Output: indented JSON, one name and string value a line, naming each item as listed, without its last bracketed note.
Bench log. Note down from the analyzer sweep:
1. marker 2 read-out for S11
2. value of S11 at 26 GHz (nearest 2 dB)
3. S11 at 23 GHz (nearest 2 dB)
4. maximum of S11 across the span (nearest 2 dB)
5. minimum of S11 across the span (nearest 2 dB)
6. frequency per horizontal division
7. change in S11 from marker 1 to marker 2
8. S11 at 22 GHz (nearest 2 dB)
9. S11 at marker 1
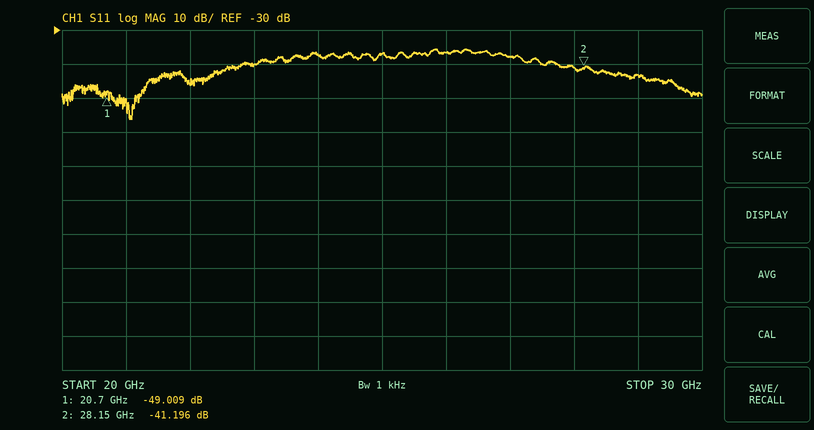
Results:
{
  "marker 2 read-out for S11": "-41.196 dB",
  "value of S11 at 26 GHz": "-36 dB",
  "S11 at 23 GHz": "-40 dB",
  "maximum of S11 across the span": "-36 dB",
  "minimum of S11 across the span": "-56 dB",
  "frequency per horizontal division": "1 GHz",
  "change in S11 from marker 1 to marker 2": "7.813 dB",
  "S11 at 22 GHz": "-46 dB",
  "S11 at marker 1": "-49.009 dB"
}
